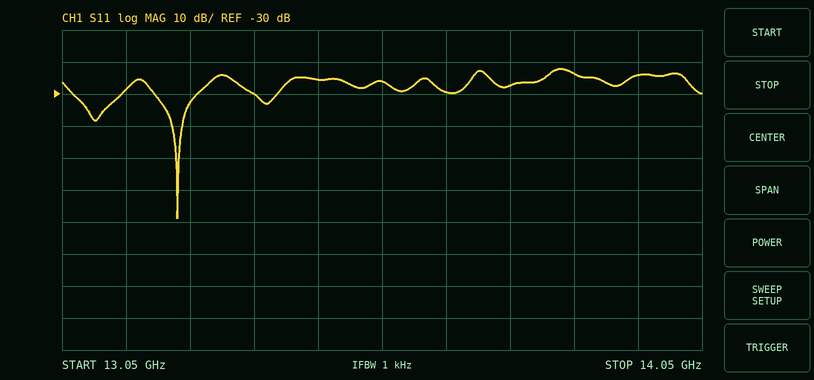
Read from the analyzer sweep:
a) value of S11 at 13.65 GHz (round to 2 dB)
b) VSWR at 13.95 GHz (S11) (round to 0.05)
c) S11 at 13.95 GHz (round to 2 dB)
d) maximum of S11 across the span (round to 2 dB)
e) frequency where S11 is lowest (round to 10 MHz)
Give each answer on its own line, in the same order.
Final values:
-30 dB
1.15
-24 dB
-22 dB
13.23 GHz
